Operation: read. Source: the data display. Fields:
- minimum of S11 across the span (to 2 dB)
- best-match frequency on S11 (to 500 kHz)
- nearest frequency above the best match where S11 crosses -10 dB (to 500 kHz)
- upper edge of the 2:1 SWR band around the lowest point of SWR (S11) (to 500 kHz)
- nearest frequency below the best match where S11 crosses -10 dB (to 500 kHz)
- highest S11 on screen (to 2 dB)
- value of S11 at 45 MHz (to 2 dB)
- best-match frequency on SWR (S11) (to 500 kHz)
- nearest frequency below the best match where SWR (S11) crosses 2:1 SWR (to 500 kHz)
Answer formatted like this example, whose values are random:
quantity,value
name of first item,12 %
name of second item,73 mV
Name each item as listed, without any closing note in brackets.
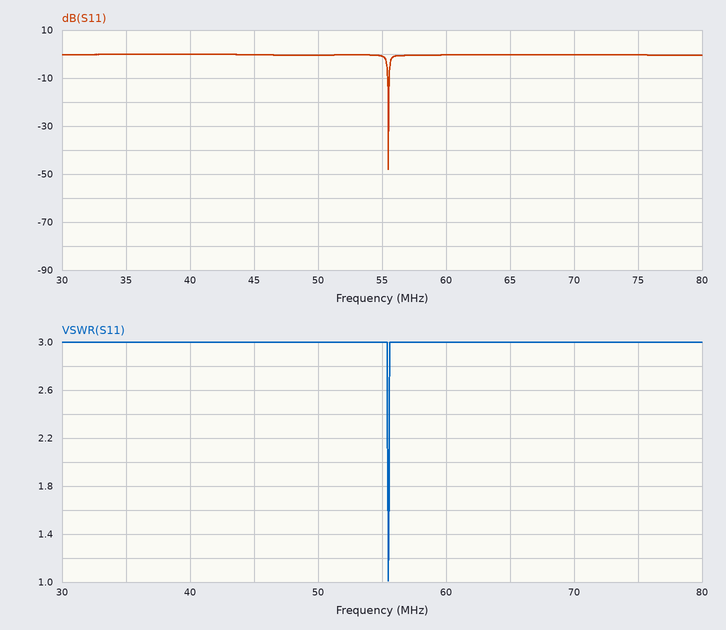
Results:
quantity,value
minimum of S11 across the span,-48 dB
best-match frequency on S11,55.5 MHz
nearest frequency above the best match where S11 crosses -10 dB,55.5 MHz
upper edge of the 2:1 SWR band around the lowest point of SWR (S11),55.5 MHz
nearest frequency below the best match where S11 crosses -10 dB,55.5 MHz
highest S11 on screen,0 dB
value of S11 at 45 MHz,0 dB
best-match frequency on SWR (S11),55.5 MHz
nearest frequency below the best match where SWR (S11) crosses 2:1 SWR,55.5 MHz
